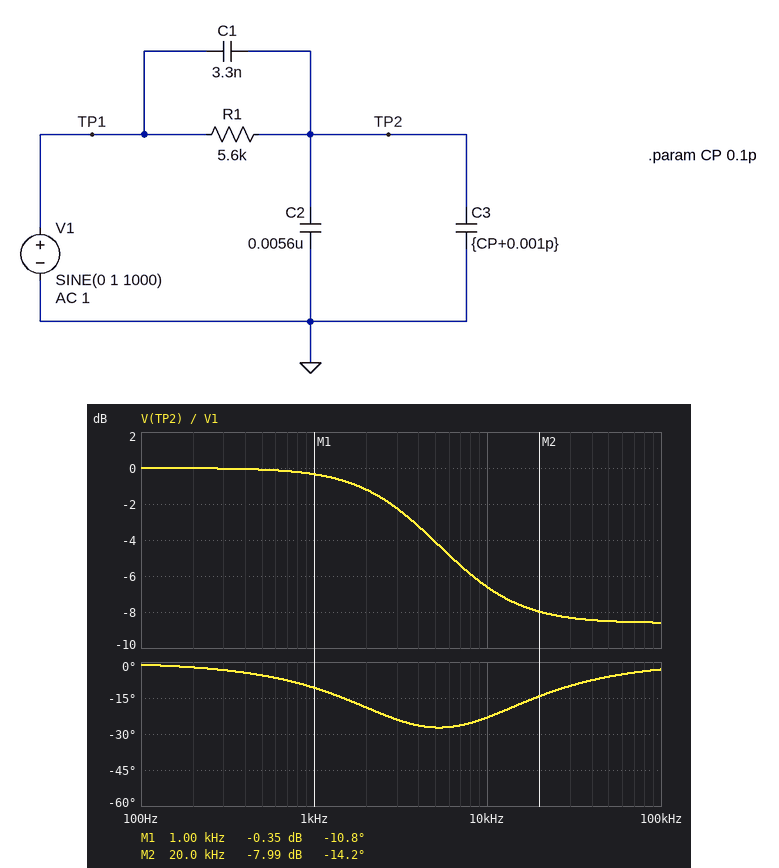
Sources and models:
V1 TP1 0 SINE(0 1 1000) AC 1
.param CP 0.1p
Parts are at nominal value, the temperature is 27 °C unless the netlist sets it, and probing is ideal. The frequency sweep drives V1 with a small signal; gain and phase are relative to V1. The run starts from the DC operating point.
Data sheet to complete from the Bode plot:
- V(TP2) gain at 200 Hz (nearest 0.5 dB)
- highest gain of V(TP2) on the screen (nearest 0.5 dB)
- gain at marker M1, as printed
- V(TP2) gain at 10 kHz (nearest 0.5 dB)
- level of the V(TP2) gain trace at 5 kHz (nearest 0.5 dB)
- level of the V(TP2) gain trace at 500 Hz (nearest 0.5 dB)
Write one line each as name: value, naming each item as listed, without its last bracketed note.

V(TP2) gain at 200 Hz: 0 dB
highest gain of V(TP2) on the screen: 0 dB
gain at marker M1, as printed: -0.35 dB
V(TP2) gain at 10 kHz: -6.5 dB
level of the V(TP2) gain trace at 5 kHz: -4.0 dB
level of the V(TP2) gain trace at 500 Hz: 0 dB
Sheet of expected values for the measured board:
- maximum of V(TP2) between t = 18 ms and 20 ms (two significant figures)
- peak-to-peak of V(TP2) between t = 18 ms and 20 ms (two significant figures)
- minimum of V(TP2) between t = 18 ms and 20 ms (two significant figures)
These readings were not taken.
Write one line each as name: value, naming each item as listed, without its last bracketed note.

maximum of V(TP2) between t = 18 ms and 20 ms: 960 mV
peak-to-peak of V(TP2) between t = 18 ms and 20 ms: 1.9 V
minimum of V(TP2) between t = 18 ms and 20 ms: -960 mV
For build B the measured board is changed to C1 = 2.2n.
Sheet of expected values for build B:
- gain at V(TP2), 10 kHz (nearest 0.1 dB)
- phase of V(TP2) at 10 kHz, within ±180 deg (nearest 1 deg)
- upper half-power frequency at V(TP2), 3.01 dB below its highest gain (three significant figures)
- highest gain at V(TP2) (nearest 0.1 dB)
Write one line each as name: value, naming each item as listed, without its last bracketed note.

gain at V(TP2), 10 kHz: -7.3 dB
phase of V(TP2) at 10 kHz, within ±180 deg: -32 deg
upper half-power frequency at V(TP2), 3.01 dB below its highest gain: 3.97 kHz
highest gain at V(TP2): 0 dB
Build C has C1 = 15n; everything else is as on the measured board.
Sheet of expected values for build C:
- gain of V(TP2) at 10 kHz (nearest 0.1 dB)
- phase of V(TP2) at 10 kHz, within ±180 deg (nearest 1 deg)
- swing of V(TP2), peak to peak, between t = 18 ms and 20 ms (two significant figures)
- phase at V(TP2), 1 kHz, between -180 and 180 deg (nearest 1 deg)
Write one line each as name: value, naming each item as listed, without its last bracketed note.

gain of V(TP2) at 10 kHz: -2.7 dB
phase of V(TP2) at 10 kHz, within ±180 deg: -3 deg
swing of V(TP2), peak to peak, between t = 18 ms and 20 ms: 1.8 V
phase at V(TP2), 1 kHz, between -180 and 180 deg: -8 deg
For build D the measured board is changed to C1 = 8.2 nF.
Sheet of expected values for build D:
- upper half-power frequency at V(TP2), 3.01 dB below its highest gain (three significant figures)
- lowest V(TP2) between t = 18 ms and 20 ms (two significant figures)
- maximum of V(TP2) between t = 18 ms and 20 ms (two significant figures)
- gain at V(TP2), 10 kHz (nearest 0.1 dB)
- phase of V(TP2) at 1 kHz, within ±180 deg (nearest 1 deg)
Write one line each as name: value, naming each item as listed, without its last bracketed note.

upper half-power frequency at V(TP2), 3.01 dB below its highest gain: 3.80 kHz
lowest V(TP2) between t = 18 ms and 20 ms: -940 mV
maximum of V(TP2) between t = 18 ms and 20 ms: 940 mV
gain at V(TP2), 10 kHz: -4.2 dB
phase of V(TP2) at 1 kHz, within ±180 deg: -10 deg
